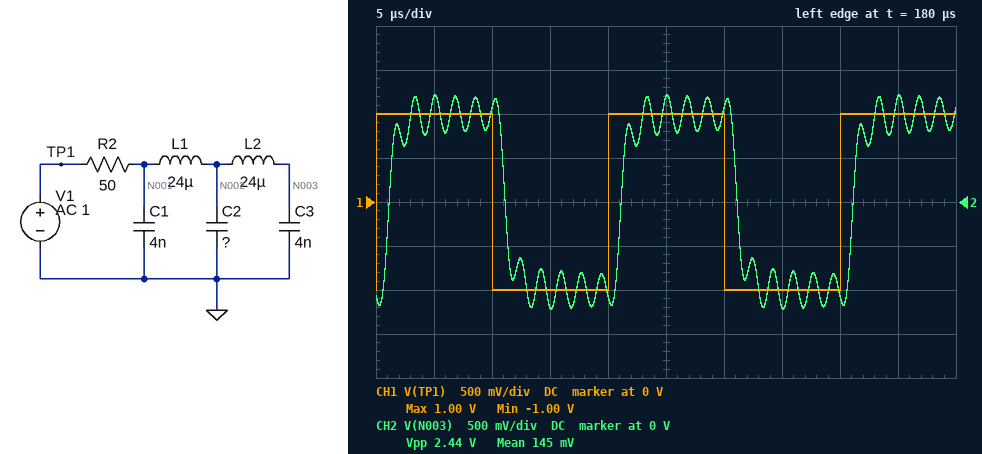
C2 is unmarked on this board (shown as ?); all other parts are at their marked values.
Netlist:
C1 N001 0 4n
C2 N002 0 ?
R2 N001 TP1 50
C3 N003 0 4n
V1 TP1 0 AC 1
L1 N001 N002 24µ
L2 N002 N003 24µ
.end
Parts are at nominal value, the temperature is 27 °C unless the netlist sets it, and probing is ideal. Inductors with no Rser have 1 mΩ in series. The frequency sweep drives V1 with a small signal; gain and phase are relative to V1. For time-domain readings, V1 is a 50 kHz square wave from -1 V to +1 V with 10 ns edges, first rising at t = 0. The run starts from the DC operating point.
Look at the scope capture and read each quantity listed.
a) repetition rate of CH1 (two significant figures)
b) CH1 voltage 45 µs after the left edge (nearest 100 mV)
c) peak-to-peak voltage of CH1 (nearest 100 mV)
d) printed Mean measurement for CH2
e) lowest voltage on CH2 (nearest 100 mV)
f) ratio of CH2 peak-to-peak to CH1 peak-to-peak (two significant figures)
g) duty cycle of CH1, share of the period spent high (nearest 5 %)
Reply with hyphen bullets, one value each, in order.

- 50 kHz
- 1.0 V
- 2.0 V
- 145 mV
- -1.2 V
- 1.2
- 50 %
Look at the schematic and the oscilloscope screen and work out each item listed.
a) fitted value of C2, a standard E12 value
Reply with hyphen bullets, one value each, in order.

- 18 nF
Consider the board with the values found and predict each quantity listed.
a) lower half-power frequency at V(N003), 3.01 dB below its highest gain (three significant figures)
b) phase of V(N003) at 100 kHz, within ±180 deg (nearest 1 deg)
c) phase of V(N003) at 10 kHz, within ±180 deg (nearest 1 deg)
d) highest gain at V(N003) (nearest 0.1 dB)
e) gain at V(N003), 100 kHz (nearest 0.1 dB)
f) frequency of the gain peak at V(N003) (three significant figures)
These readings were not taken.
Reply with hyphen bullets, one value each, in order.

- 572 kHz
- -45 deg
- -5 deg
- 16.2 dB
- -0.7 dB
- 579 kHz
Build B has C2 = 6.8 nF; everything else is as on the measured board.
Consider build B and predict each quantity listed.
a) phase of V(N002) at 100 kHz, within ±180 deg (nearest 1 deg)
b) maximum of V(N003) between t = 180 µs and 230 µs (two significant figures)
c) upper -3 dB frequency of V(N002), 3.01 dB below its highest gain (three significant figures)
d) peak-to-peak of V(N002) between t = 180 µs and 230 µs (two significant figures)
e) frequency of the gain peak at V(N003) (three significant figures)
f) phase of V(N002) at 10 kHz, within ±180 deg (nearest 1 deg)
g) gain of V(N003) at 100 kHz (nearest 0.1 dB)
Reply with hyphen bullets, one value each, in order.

- -27 deg
- 1.6 V
- 739 kHz
- 2.8 V
- 709 kHz
- -3 deg
- 0.3 dB
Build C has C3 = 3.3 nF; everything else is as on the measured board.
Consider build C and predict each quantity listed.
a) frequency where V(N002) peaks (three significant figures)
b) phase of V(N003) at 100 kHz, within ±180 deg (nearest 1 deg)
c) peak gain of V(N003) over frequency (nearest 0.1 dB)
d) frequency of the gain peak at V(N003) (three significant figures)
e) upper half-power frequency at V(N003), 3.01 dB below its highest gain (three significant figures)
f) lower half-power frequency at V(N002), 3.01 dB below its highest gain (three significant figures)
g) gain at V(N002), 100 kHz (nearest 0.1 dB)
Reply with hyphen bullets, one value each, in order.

- 625 kHz
- -44 deg
- 18.9 dB
- 624 kHz
- 629 kHz
- 620 kHz
- -0.9 dB
